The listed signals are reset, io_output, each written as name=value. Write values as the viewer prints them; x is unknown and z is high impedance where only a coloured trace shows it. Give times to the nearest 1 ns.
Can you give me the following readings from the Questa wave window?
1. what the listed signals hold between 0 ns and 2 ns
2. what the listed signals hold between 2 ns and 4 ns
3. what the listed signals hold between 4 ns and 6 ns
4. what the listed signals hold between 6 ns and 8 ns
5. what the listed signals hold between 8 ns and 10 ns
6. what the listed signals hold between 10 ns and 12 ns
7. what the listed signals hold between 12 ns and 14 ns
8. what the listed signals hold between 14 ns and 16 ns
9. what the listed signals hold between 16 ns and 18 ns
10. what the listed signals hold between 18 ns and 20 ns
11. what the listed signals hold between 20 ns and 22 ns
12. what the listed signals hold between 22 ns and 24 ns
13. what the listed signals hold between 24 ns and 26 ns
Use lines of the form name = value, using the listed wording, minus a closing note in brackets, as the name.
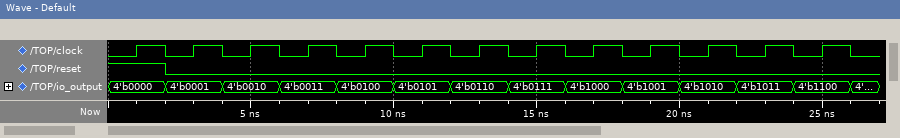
what the listed signals hold between 0 ns and 2 ns = reset=1, io_output=4'b0000
what the listed signals hold between 2 ns and 4 ns = reset=0, io_output=4'b0001
what the listed signals hold between 4 ns and 6 ns = reset=0, io_output=4'b0010
what the listed signals hold between 6 ns and 8 ns = reset=0, io_output=4'b0011
what the listed signals hold between 8 ns and 10 ns = reset=0, io_output=4'b0100
what the listed signals hold between 10 ns and 12 ns = reset=0, io_output=4'b0101
what the listed signals hold between 12 ns and 14 ns = reset=0, io_output=4'b0110
what the listed signals hold between 14 ns and 16 ns = reset=0, io_output=4'b0111
what the listed signals hold between 16 ns and 18 ns = reset=0, io_output=4'b1000
what the listed signals hold between 18 ns and 20 ns = reset=0, io_output=4'b1001
what the listed signals hold between 20 ns and 22 ns = reset=0, io_output=4'b1010
what the listed signals hold between 22 ns and 24 ns = reset=0, io_output=4'b1011
what the listed signals hold between 24 ns and 26 ns = reset=0, io_output=4'b1100
